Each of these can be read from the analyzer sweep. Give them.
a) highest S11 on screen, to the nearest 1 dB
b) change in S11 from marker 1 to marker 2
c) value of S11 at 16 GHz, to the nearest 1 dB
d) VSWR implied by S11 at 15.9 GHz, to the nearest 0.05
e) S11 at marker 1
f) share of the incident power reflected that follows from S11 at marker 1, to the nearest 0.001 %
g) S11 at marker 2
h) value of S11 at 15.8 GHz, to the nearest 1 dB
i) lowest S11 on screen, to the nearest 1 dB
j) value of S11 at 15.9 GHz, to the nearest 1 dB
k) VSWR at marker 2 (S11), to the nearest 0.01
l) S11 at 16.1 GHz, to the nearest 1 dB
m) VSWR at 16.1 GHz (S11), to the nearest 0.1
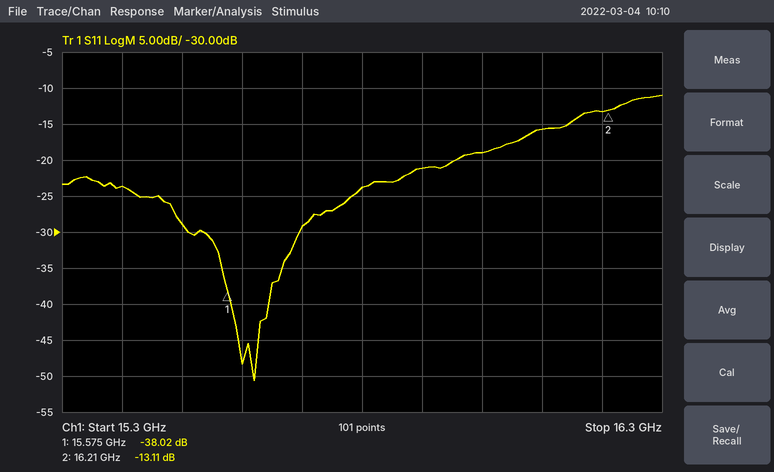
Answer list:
-11 dB
24.91 dB
-19 dB
1.20
-38.02 dB
0.016 %
-13.11 dB
-24 dB
-51 dB
-21 dB
1.57
-16 dB
1.4
